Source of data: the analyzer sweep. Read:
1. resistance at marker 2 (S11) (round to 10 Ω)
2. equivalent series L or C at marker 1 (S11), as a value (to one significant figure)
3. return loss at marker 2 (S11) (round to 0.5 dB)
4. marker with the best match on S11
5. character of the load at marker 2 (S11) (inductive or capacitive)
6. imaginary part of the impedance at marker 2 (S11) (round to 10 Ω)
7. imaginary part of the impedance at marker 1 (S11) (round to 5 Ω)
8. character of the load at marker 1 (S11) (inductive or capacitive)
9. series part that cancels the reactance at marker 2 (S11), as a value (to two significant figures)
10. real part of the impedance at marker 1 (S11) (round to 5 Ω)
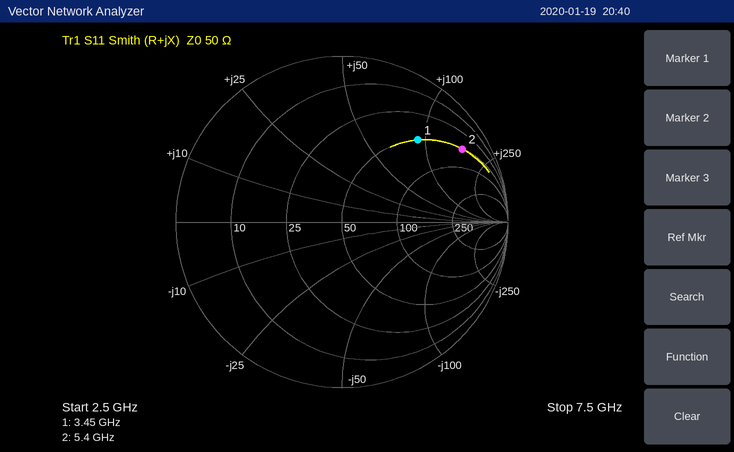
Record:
50 Ω
4 nH
1.5 dB
marker 1
inductive
+160 Ω
+90 Ω
inductive
180 fF
50 Ω
